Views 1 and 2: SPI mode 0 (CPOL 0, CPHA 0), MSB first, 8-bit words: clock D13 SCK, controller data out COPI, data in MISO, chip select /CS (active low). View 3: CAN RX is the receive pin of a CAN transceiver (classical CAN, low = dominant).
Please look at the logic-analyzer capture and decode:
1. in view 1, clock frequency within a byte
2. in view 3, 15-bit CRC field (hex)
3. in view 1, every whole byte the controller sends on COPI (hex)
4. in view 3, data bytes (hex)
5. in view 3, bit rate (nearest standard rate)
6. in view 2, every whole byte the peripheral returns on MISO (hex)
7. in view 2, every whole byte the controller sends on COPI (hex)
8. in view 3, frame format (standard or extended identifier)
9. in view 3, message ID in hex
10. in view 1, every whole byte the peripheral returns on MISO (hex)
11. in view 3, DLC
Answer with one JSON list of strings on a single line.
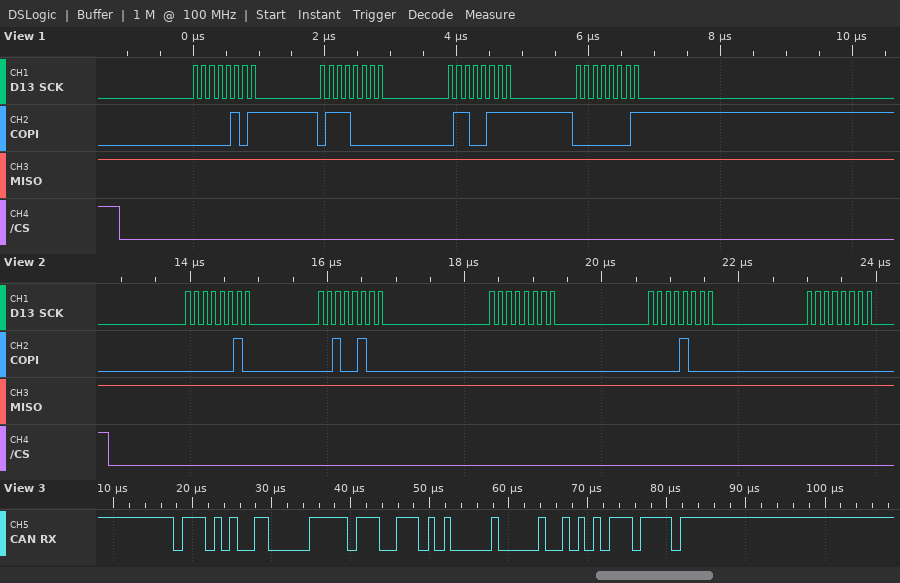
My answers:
["8 MHz", "0x1577", "0x05 0x70 0x67 0x01", "F9 D4 00", "1000 kbit/s", "0xFF 0xFF 0xFF 0xFF 0xFF", "0x02 0x24 0x00 0x08 0x00", "standard", "0x753", "0xFF 0xFF 0xFF 0xFF", "3"]
